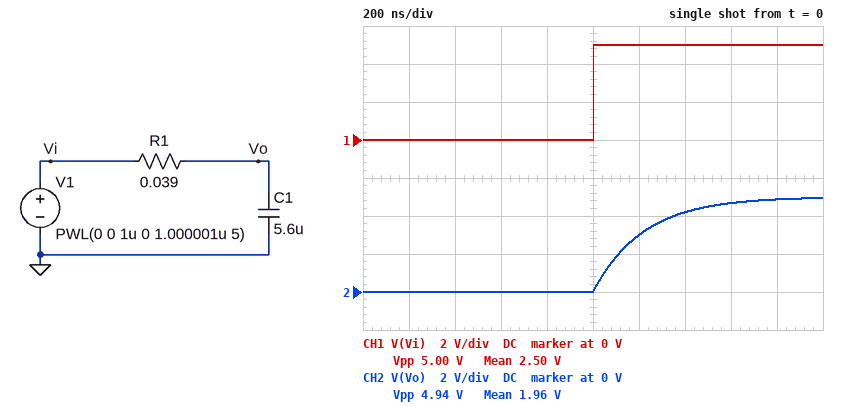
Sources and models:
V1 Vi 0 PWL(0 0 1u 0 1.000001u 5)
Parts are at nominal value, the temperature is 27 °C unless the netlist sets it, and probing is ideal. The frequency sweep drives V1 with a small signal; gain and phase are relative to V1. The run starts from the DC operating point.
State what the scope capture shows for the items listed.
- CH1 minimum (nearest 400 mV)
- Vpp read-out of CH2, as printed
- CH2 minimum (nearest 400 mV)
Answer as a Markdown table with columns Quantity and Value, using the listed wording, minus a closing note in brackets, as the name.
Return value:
| Quantity | Value |
|---|---|
| CH1 minimum | 0 V |
| Vpp read-out of CH2, as printed | 4.94 V |
| CH2 minimum | 0 V |
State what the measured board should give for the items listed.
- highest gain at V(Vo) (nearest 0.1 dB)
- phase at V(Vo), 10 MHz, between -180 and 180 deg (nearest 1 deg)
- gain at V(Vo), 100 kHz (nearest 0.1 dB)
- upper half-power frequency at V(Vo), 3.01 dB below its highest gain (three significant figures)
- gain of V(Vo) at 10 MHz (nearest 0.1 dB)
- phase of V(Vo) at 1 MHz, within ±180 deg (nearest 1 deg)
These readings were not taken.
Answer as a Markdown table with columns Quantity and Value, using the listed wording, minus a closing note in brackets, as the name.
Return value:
| Quantity | Value |
|---|---|
| highest gain at V(Vo) | 0 dB |
| phase at V(Vo), 10 MHz, between -180 and 180 deg | -86 deg |
| gain at V(Vo), 100 kHz | -0.1 dB |
| upper half-power frequency at V(Vo), 3.01 dB below its highest gain | 729 kHz |
| gain of V(Vo) at 10 MHz | -22.8 dB |
| phase of V(Vo) at 1 MHz, within ±180 deg | -54 deg |
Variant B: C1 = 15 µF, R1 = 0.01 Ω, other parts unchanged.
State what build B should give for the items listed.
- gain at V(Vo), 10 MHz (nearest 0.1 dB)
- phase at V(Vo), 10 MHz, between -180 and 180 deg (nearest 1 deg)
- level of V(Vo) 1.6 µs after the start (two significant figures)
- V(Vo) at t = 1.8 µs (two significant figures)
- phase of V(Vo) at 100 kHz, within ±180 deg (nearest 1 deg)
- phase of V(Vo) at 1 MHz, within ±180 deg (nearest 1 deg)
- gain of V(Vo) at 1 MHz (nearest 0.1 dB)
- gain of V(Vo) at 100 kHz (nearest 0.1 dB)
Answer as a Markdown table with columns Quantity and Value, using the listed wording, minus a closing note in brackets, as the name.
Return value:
| Quantity | Value |
|---|---|
| gain at V(Vo), 10 MHz | -19.5 dB |
| phase at V(Vo), 10 MHz, between -180 and 180 deg | -84 deg |
| level of V(Vo) 1.6 µs after the start | 4.9 V |
| V(Vo) at t = 1.8 µs | 5.0 V |
| phase of V(Vo) at 100 kHz, within ±180 deg | -5 deg |
| phase of V(Vo) at 1 MHz, within ±180 deg | -43 deg |
| gain of V(Vo) at 1 MHz | -2.8 dB |
| gain of V(Vo) at 100 kHz | 0 dB |
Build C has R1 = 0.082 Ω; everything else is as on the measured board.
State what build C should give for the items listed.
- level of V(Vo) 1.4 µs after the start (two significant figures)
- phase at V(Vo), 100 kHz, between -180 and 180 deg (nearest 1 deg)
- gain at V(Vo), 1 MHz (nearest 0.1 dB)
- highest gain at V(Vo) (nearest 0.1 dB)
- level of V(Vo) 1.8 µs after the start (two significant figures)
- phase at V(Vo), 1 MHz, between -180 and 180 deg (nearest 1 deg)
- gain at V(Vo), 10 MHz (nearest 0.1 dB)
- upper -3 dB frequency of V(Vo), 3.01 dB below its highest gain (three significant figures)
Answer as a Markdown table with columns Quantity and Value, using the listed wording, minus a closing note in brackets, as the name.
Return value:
| Quantity | Value |
|---|---|
| level of V(Vo) 1.4 µs after the start | 2.9 V |
| phase at V(Vo), 100 kHz, between -180 and 180 deg | -16 deg |
| gain at V(Vo), 1 MHz | -9.7 dB |
| highest gain at V(Vo) | 0 dB |
| level of V(Vo) 1.8 µs after the start | 4.1 V |
| phase at V(Vo), 1 MHz, between -180 and 180 deg | -71 deg |
| gain at V(Vo), 10 MHz | -29.2 dB |
| upper -3 dB frequency of V(Vo), 3.01 dB below its highest gain | 347 kHz |
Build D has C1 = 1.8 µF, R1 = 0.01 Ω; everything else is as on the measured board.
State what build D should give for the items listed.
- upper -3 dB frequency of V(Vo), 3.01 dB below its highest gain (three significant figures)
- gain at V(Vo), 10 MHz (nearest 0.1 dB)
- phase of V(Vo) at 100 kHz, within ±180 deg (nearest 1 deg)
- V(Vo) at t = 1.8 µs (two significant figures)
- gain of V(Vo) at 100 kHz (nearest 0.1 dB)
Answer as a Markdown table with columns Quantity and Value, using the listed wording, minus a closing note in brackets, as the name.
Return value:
| Quantity | Value |
|---|---|
| upper -3 dB frequency of V(Vo), 3.01 dB below its highest gain | 8.84 MHz |
| gain at V(Vo), 10 MHz | -3.6 dB |
| phase of V(Vo) at 100 kHz, within ±180 deg | -1 deg |
| V(Vo) at t = 1.8 µs | 5.0 V |
| gain of V(Vo) at 100 kHz | 0 dB |
